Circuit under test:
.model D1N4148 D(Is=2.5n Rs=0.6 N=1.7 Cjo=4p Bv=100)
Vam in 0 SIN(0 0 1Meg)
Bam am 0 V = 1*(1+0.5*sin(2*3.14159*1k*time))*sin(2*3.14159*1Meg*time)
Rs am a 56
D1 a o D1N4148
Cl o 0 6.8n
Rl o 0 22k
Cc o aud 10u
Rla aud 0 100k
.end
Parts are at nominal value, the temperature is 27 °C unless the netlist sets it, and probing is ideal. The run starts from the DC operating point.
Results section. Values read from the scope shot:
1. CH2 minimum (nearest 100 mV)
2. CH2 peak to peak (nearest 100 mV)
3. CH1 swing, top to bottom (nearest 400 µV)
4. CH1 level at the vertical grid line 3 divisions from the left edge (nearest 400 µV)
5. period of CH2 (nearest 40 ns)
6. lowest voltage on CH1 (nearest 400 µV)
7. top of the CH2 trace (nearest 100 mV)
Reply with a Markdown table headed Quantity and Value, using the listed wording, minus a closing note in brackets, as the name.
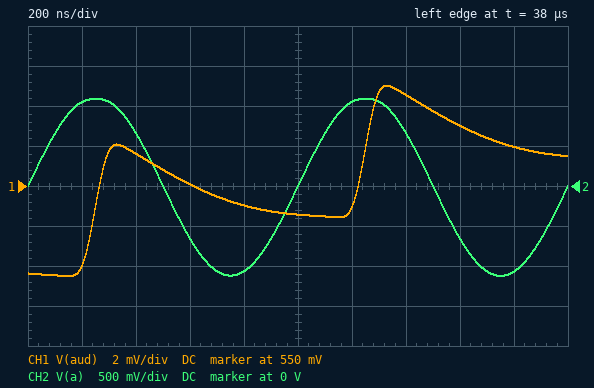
| Quantity | Value |
|---|---|
| CH2 minimum | -1.1 V |
| CH2 peak to peak | 2.2 V |
| CH1 swing, top to bottom | 9.6 mV |
| CH1 level at the vertical grid line 3 divisions from the left edge | 550.0 mV |
| period of CH2 | 1.00 µs |
| lowest voltage on CH1 | 545.6 mV |
| top of the CH2 trace | 1.1 V |
